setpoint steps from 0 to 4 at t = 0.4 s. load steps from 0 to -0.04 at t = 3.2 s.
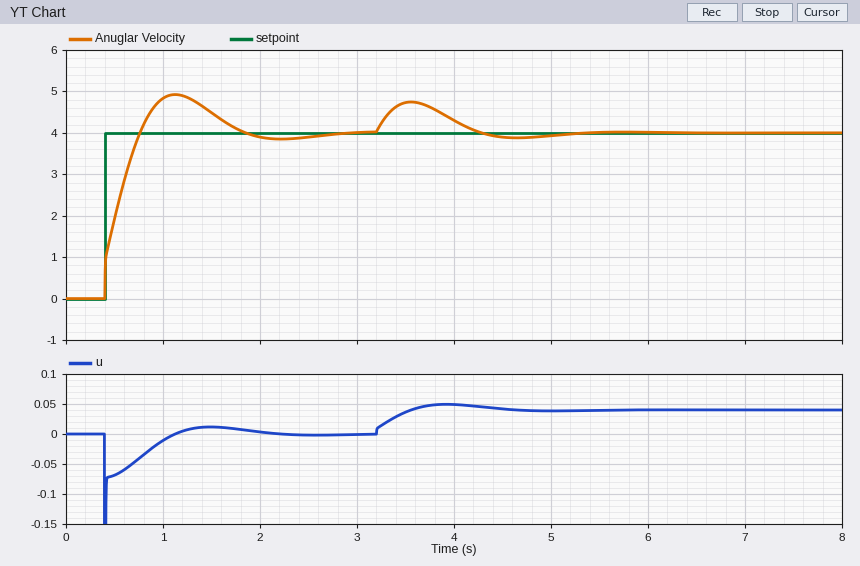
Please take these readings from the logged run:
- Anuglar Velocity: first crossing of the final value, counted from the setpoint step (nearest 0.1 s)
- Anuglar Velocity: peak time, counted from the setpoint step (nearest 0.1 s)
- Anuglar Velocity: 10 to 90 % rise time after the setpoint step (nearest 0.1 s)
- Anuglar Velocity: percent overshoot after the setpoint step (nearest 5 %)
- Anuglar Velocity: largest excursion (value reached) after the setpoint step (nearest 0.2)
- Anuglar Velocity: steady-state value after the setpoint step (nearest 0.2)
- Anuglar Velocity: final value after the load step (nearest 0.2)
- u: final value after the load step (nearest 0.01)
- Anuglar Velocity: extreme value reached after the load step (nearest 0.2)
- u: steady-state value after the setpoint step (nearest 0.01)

0.4 s
0.7 s
0.3 s
25 %
5.0
4.0
4.0
0.04
4.8
0.00
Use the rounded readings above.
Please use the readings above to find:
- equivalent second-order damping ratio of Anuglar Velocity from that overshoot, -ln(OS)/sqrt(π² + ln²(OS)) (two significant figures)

0.40
